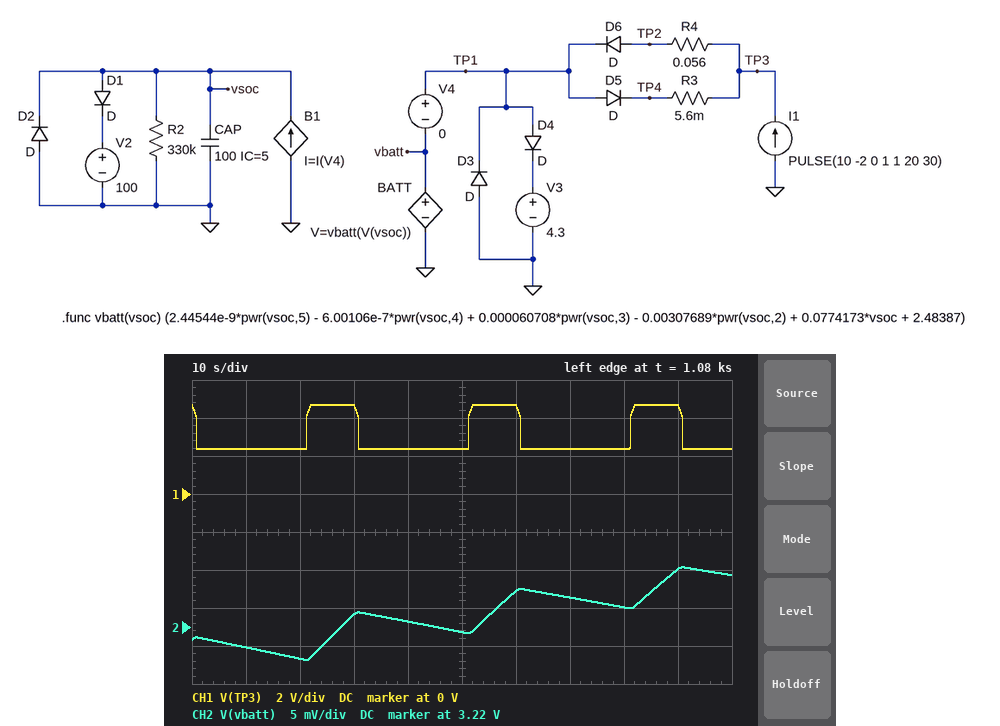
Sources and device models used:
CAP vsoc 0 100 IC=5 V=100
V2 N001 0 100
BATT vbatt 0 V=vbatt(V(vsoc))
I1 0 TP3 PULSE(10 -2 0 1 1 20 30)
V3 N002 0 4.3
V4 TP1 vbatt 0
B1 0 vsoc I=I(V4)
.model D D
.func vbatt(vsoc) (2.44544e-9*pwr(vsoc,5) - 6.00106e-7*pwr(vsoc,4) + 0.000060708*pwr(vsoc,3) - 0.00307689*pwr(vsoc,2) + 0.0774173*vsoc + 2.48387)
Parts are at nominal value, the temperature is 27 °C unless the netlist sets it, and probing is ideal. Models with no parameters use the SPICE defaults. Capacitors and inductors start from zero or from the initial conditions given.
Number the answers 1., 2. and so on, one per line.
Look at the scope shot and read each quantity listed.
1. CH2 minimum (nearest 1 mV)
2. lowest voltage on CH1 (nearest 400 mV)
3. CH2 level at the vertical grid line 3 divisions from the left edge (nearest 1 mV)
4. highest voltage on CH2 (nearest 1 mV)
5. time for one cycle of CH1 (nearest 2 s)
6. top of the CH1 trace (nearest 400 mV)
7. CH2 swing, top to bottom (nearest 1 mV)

1. 3.216 V
2. 2.4 V
3. 3.222 V
4. 3.228 V
5. 30 s
6. 4.8 V
7. 12 mV
